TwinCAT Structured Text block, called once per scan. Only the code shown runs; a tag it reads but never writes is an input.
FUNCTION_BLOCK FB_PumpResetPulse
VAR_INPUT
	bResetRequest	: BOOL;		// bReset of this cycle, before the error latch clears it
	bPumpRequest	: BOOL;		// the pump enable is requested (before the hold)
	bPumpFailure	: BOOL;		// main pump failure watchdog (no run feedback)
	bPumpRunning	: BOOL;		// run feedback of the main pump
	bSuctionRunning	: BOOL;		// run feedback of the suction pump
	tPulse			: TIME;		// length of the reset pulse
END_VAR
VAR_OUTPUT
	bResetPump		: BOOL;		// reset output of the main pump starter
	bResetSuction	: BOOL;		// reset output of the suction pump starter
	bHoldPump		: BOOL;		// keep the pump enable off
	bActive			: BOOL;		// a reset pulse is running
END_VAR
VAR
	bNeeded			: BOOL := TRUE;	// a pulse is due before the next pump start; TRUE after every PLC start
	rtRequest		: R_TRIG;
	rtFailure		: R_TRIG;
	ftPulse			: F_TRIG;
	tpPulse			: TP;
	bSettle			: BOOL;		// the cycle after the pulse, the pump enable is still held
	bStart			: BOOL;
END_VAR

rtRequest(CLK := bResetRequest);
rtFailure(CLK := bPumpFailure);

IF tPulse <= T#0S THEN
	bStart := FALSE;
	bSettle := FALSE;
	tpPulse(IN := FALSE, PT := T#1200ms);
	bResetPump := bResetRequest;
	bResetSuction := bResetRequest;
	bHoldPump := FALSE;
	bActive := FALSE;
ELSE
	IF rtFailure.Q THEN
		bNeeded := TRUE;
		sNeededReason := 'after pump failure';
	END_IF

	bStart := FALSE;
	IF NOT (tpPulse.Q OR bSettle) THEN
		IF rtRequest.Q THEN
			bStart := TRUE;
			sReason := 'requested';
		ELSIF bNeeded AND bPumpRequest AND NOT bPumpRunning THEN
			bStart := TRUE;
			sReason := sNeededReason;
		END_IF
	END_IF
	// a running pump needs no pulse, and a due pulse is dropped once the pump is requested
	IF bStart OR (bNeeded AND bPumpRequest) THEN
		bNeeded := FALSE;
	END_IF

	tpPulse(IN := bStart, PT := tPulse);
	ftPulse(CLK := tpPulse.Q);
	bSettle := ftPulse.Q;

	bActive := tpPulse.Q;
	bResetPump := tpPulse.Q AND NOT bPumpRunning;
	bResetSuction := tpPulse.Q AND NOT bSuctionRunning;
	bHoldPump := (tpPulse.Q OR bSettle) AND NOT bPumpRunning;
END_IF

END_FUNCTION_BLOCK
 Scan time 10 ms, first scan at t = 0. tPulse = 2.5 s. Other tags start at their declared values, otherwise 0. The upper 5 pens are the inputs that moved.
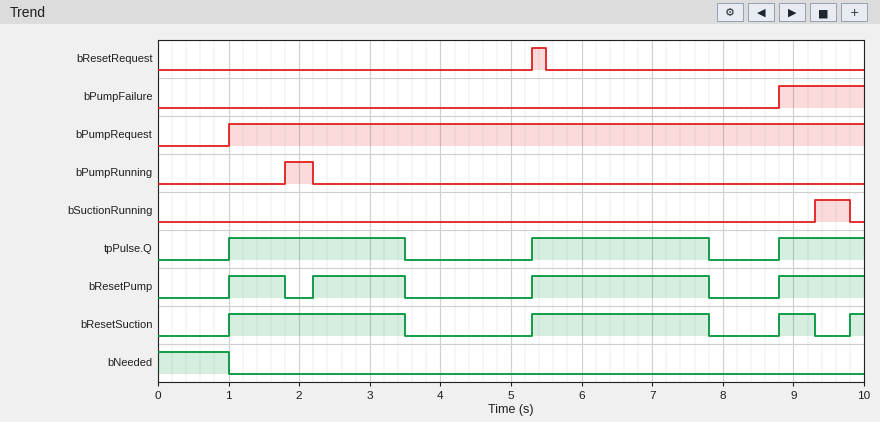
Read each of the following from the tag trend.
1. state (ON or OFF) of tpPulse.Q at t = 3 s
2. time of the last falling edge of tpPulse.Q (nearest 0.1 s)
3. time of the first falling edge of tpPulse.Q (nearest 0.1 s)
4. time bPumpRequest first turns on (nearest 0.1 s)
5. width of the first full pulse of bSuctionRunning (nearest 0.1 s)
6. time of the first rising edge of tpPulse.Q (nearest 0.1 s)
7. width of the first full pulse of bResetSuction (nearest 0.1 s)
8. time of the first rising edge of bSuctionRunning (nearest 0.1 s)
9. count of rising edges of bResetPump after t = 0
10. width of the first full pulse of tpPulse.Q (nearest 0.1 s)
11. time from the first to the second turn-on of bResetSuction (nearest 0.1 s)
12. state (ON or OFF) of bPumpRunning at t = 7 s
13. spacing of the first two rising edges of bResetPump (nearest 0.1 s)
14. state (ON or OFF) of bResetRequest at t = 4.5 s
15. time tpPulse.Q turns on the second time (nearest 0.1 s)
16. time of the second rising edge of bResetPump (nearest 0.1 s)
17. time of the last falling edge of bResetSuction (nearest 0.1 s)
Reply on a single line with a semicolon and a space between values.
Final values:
ON; 7.8 s; 3.5 s; 1.0 s; 0.5 s; 1.0 s; 2.5 s; 9.3 s; 4; 2.5 s; 4.3 s; OFF; 1.2 s; OFF; 5.3 s; 2.2 s; 9.3 s
